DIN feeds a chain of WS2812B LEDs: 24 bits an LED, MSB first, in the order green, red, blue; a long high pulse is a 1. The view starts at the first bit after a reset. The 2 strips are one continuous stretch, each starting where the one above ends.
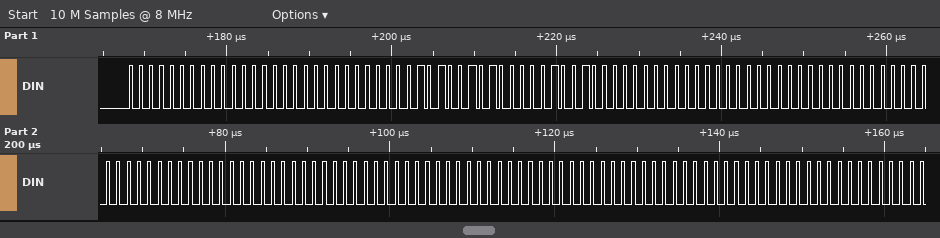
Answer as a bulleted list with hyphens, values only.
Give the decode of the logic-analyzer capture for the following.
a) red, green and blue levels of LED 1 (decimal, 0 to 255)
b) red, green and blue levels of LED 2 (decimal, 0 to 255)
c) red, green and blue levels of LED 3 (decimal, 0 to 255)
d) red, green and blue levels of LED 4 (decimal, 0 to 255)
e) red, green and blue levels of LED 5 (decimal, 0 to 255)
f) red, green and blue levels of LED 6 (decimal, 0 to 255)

- 0, 0, 0
- 80, 10, 72
- 0, 0, 0
- 0, 0, 0
- 0, 0, 0
- 0, 0, 0
